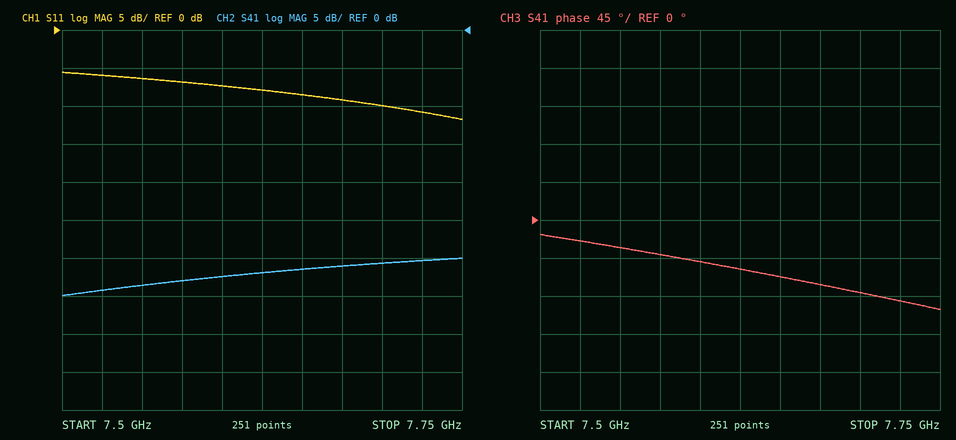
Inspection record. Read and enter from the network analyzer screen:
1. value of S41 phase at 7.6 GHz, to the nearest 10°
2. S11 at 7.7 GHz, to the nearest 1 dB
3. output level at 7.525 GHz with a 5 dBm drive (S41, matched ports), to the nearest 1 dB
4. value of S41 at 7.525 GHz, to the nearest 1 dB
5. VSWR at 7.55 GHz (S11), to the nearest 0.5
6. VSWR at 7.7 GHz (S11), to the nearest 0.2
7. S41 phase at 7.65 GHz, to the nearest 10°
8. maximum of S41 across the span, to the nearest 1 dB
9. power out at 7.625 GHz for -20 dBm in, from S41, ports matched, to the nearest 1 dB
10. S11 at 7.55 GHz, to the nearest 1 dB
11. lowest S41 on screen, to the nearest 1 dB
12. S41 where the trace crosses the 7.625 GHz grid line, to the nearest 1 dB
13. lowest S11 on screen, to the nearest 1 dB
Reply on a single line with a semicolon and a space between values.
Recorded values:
-50°; -10 dB; -29 dBm; -34 dB; 3.0; 2.0; -70°; -30 dB; -52 dBm; -6 dB; -35 dB; -32 dB; -12 dB
